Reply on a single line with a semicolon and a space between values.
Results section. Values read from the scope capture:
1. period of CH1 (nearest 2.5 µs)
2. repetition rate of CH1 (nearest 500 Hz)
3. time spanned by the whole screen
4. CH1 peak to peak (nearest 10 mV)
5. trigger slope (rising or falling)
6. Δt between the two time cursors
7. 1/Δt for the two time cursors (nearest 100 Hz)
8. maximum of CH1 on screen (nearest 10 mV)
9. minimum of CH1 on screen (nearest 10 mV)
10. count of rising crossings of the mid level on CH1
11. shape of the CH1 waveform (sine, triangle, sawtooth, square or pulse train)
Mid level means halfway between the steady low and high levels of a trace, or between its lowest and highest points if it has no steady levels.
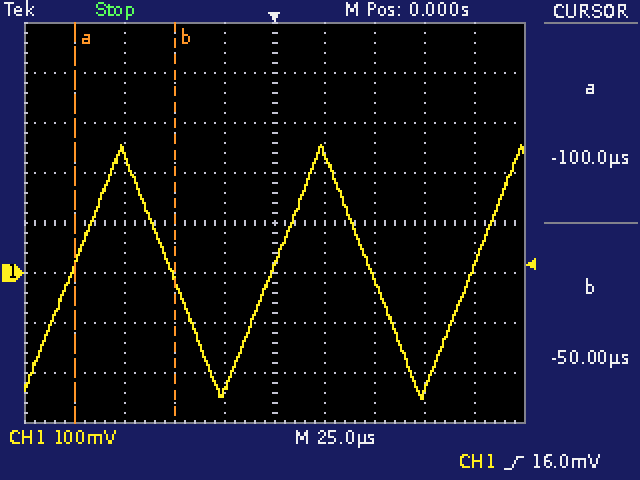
100.0 µs; 10.0 kHz; 250 µs; 510 mV; rising; 50.0 µs; 20.0 kHz; 260 mV; -250 mV; 3; triangle
